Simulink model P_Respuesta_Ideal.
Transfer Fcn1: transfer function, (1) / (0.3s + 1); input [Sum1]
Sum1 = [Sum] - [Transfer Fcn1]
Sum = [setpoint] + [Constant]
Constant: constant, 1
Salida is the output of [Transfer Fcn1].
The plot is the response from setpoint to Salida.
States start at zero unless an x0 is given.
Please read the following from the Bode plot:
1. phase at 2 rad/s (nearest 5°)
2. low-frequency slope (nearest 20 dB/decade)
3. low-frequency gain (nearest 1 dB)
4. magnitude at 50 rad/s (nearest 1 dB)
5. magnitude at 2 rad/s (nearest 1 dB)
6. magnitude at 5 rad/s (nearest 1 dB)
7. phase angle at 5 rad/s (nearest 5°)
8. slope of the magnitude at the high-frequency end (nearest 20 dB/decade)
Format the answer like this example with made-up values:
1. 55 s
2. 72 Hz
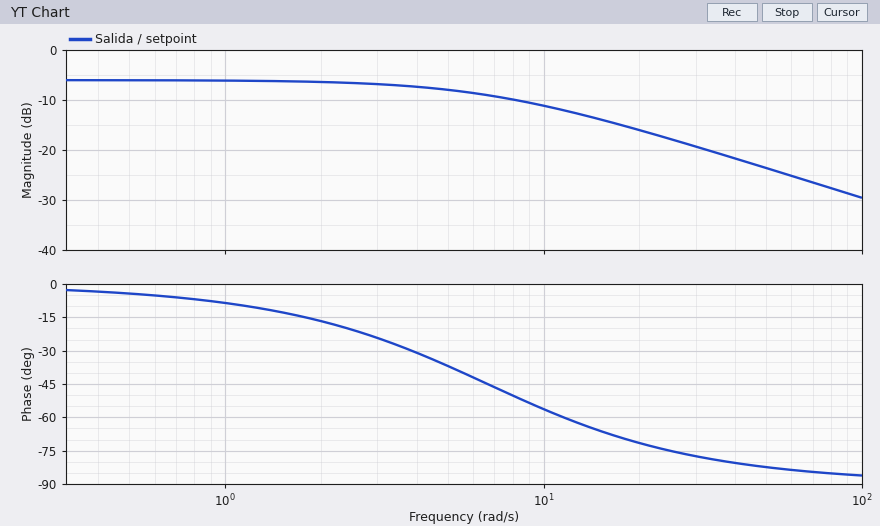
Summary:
1. -15°
2. 0 dB/decade
3. -6 dB
4. -24 dB
5. -6 dB
6. -8 dB
7. -35°
8. -20 dB/decade
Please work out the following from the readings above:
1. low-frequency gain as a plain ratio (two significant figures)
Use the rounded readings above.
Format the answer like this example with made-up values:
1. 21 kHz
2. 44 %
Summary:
1. 0.50
